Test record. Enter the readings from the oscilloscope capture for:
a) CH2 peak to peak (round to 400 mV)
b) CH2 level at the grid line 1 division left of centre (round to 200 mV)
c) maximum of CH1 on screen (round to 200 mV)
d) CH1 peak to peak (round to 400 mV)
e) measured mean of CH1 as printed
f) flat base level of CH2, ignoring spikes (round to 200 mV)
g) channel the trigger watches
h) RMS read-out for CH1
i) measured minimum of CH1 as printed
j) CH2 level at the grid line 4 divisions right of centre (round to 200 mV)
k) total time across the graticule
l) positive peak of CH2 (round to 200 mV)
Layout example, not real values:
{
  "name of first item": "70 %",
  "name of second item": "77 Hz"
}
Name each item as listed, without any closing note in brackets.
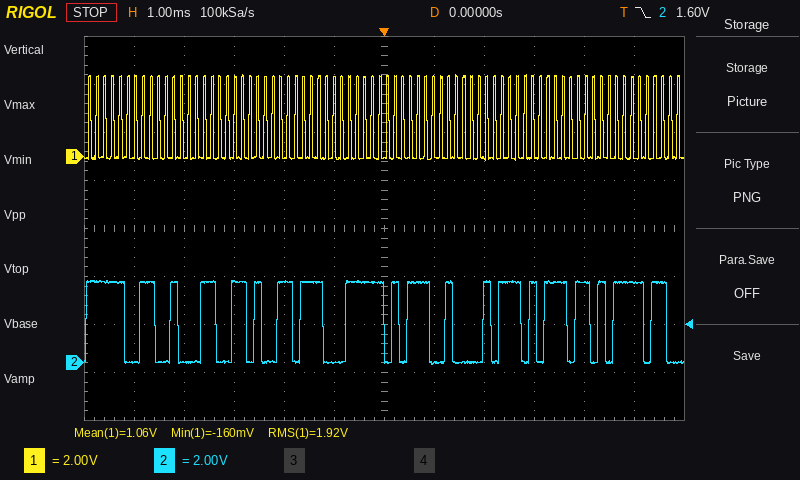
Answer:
{
  "CH2 peak to peak": "3.6 V",
  "CH2 level at the grid line 1 division left of centre": "0.0 V",
  "maximum of CH1 on screen": "3.4 V",
  "CH1 peak to peak": "3.6 V",
  "measured mean of CH1 as printed": "1.06 V",
  "flat base level of CH2, ignoring spikes": "0.0 V",
  "channel the trigger watches": "CH2",
  "RMS read-out for CH1": "1.92 V",
  "measured minimum of CH1 as printed": "-160 mV",
  "CH2 level at the grid line 4 divisions right of centre": "3.4 V",
  "total time across the graticule": "12 ms",
  "positive peak of CH2": "3.4 V"
}
